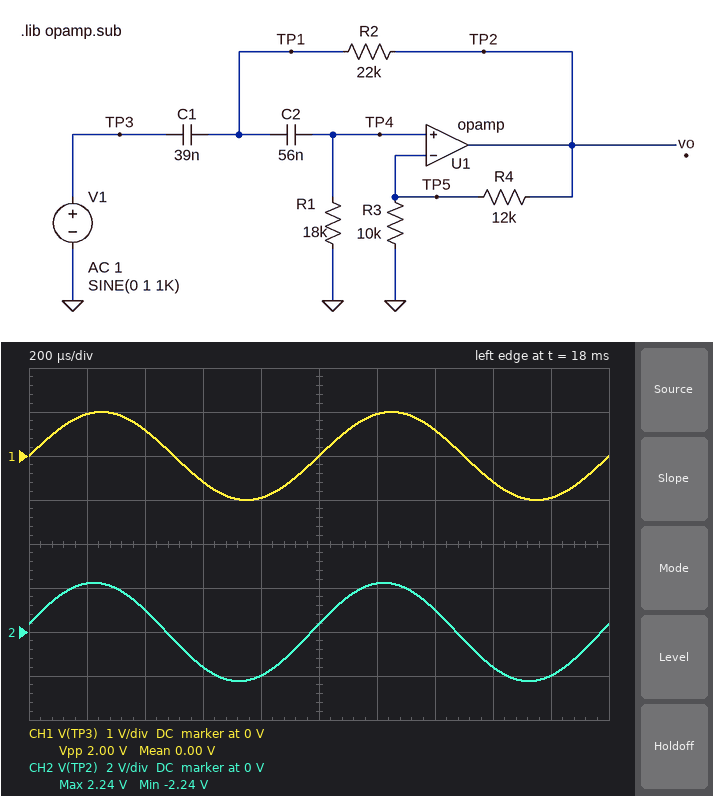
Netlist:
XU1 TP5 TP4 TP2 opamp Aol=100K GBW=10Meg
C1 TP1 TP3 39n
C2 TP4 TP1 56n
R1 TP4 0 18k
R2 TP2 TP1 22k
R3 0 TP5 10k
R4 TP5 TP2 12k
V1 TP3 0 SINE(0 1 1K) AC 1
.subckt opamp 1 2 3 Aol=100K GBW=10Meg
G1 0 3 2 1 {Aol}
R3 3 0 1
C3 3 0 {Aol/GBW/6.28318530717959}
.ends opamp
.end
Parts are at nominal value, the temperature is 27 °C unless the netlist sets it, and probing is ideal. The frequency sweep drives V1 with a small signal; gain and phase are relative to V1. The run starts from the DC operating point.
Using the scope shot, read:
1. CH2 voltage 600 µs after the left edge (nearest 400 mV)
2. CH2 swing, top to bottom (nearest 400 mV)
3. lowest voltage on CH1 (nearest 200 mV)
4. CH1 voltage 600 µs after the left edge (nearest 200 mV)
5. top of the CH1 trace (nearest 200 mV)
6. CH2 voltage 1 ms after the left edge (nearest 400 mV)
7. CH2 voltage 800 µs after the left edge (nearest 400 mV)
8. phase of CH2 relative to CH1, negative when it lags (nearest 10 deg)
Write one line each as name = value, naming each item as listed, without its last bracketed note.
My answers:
CH2 voltage 600 µs after the left edge = -1.6 V
CH2 swing, top to bottom = 4.4 V
lowest voltage on CH1 = -1.0 V
CH1 voltage 600 µs after the left edge = -600 mV
top of the CH1 trace = 1.0 V
CH2 voltage 1 ms after the left edge = 400 mV
CH2 voltage 800 µs after the left edge = -2.0 V
phase of CH2 relative to CH1, negative when it lags = 10 deg
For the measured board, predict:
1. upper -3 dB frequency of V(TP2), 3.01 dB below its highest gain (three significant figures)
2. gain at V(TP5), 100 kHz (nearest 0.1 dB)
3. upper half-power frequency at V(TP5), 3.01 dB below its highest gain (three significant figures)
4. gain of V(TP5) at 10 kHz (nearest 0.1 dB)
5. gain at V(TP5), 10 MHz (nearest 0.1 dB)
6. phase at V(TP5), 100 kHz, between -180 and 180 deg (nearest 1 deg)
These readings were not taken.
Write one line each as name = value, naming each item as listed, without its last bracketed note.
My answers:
upper -3 dB frequency of V(TP2), 3.01 dB below its highest gain = 2.84 MHz
gain at V(TP5), 100 kHz = 0 dB
upper half-power frequency at V(TP5), 3.01 dB below its highest gain = 2.84 MHz
gain of V(TP5) at 10 kHz = 0 dB
gain at V(TP5), 10 MHz = -7.7 dB
phase at V(TP5), 100 kHz, between -180 and 180 deg = -1 deg
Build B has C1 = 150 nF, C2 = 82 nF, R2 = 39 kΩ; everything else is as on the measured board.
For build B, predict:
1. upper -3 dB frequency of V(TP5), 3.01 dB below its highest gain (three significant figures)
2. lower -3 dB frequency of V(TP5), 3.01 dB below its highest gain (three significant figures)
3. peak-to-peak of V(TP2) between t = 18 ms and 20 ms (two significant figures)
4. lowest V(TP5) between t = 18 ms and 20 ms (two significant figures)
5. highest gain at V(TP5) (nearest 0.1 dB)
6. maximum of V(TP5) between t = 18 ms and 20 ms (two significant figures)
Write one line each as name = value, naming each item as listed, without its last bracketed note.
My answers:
upper -3 dB frequency of V(TP5), 3.01 dB below its highest gain = 4.55 MHz
lower -3 dB frequency of V(TP5), 3.01 dB below its highest gain = 113 Hz
peak-to-peak of V(TP2) between t = 18 ms and 20 ms = 4.4 V
lowest V(TP5) between t = 18 ms and 20 ms = -990 mV
highest gain at V(TP5) = 0 dB
maximum of V(TP5) between t = 18 ms and 20 ms = 990 mV
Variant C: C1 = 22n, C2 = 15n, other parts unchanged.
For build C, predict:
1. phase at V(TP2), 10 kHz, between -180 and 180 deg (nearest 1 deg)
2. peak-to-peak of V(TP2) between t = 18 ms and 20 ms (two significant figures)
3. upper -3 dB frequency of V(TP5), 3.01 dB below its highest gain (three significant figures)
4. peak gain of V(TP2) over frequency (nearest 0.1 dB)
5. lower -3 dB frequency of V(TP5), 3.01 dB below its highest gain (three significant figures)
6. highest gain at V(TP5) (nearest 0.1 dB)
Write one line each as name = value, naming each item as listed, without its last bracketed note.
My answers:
phase at V(TP2), 10 kHz, between -180 and 180 deg = 3 deg
peak-to-peak of V(TP2) between t = 18 ms and 20 ms = 4.4 V
upper -3 dB frequency of V(TP5), 3.01 dB below its highest gain = 4.52 MHz
peak gain of V(TP2) over frequency = 6.9 dB
lower -3 dB frequency of V(TP5), 3.01 dB below its highest gain = 424 Hz
highest gain at V(TP5) = 0 dB
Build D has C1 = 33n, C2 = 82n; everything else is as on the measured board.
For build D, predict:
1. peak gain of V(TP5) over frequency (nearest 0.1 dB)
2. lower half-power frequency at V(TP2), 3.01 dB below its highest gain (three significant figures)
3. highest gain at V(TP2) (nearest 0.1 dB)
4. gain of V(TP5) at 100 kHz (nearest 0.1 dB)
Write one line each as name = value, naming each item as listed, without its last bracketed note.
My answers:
peak gain of V(TP5) over frequency = 3.3 dB
lower half-power frequency at V(TP2), 3.01 dB below its highest gain = 129 Hz
highest gain at V(TP2) = 10.2 dB
gain of V(TP5) at 100 kHz = 0 dB
